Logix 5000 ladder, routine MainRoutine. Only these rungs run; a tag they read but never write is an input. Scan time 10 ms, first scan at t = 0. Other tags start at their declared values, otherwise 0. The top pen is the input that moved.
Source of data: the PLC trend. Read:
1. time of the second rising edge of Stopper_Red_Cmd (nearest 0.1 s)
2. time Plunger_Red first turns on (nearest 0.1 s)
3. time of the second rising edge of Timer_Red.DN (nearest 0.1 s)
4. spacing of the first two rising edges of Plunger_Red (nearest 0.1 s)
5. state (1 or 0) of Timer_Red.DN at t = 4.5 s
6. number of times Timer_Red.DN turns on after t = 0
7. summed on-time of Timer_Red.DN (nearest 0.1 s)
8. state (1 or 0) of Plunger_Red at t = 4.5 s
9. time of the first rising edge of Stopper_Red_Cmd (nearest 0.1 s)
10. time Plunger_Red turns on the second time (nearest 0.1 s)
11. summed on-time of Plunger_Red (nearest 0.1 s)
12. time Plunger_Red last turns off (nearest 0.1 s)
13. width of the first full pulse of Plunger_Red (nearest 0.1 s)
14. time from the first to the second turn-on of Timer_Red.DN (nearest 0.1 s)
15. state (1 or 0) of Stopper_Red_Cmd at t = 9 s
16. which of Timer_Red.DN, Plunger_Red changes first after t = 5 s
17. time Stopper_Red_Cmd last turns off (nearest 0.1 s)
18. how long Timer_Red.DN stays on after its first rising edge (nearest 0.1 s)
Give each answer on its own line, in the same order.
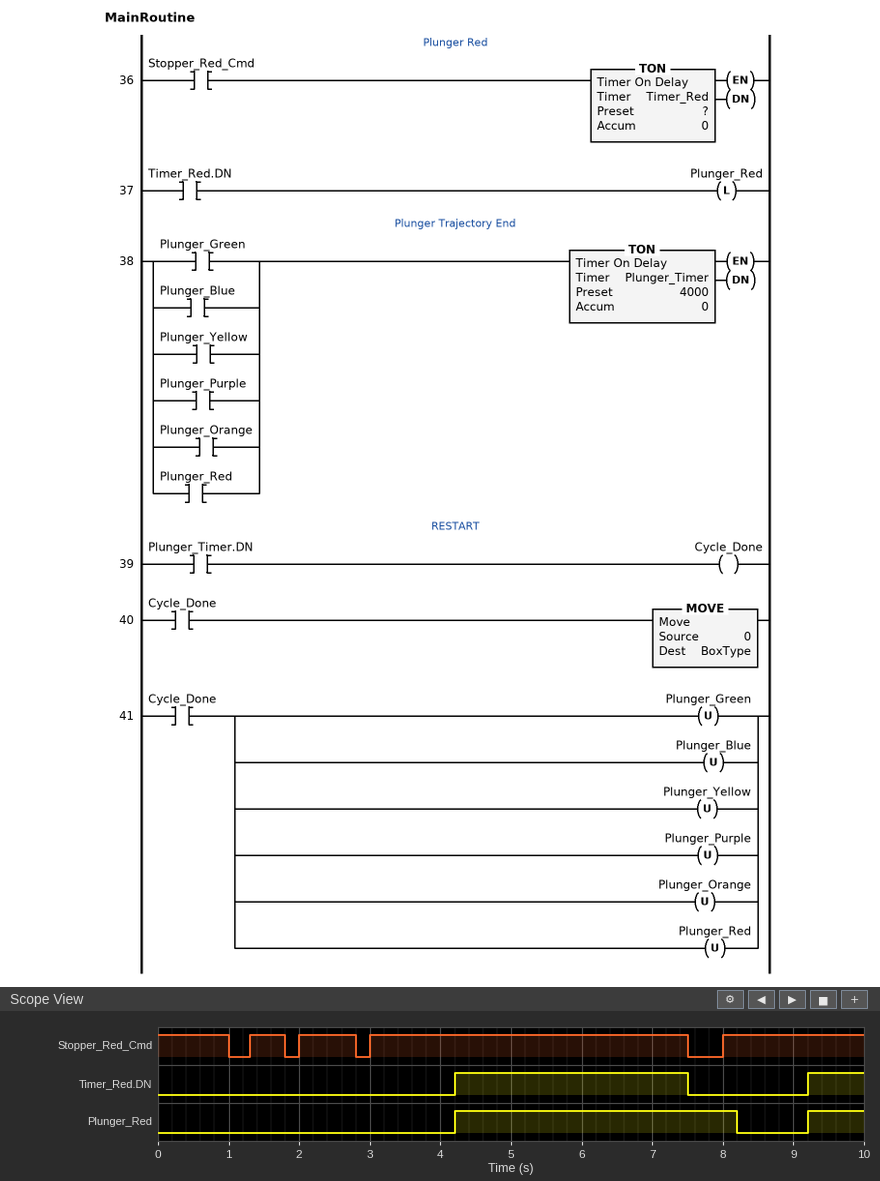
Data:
2.0 s
4.2 s
9.2 s
5.0 s
1
2
4.1 s
1
1.3 s
9.2 s
4.8 s
8.2 s
4.0 s
5.0 s
1
Timer_Red.DN
7.5 s
3.3 s
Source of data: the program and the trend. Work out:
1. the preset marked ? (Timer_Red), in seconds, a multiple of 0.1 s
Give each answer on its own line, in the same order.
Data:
1.2 s
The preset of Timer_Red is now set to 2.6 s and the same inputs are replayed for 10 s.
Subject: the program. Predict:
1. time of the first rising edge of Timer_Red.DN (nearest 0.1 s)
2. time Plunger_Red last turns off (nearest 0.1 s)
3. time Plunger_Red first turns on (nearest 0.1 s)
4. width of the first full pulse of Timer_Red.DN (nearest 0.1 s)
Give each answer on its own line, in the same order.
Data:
5.6 s
9.6 s
5.6 s
1.9 s
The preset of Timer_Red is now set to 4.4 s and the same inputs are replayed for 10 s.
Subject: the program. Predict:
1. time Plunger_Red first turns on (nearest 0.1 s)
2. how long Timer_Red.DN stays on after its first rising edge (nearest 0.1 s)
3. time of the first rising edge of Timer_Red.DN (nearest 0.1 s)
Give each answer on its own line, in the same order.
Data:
7.4 s
0.1 s
7.4 s
